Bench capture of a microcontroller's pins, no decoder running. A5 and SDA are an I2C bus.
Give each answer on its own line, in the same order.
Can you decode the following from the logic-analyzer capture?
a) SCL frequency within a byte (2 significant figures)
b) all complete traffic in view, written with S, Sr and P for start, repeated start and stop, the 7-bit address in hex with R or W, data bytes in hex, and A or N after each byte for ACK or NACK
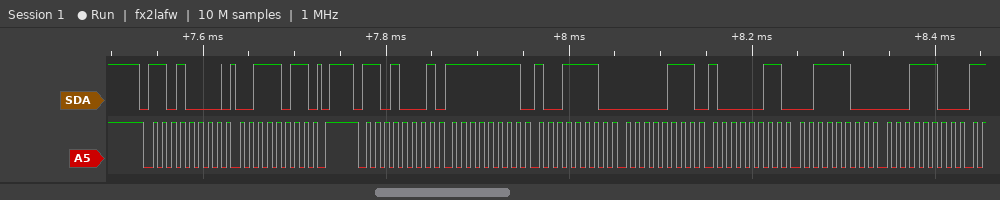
100 kHz
S 68W A 3B A P S 68R A FF A 9E A 07 A 83 A 3C A 1C A
